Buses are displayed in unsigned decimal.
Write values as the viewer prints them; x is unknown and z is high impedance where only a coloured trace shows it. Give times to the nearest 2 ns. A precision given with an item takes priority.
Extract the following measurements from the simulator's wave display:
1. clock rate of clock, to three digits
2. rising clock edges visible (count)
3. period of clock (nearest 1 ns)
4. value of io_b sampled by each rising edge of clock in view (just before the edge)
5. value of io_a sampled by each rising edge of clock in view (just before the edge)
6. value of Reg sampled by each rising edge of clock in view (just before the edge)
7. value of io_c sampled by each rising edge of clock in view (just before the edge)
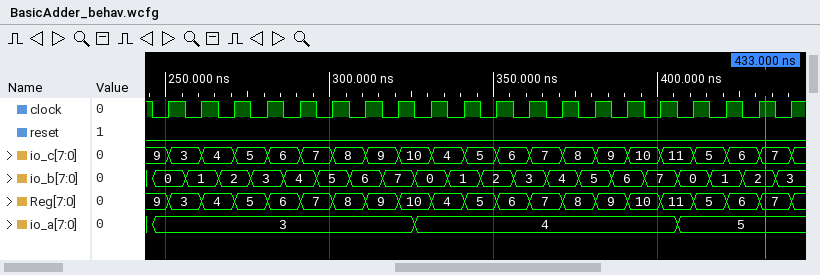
100 MHz
20
10 ns
0, 1, 2, 3, 4, 5, 6, 7, 0, 1, 2, 3, 4, 5, 6, 7, 0, 1, 2, 3
3, 3, 3, 3, 3, 3, 3, 3, 4, 4, 4, 4, 4, 4, 4, 4, 5, 5, 5, 5
9, 3, 4, 5, 6, 7, 8, 9, 10, 4, 5, 6, 7, 8, 9, 10, 11, 5, 6, 7
9, 3, 4, 5, 6, 7, 8, 9, 10, 4, 5, 6, 7, 8, 9, 10, 11, 5, 6, 7
